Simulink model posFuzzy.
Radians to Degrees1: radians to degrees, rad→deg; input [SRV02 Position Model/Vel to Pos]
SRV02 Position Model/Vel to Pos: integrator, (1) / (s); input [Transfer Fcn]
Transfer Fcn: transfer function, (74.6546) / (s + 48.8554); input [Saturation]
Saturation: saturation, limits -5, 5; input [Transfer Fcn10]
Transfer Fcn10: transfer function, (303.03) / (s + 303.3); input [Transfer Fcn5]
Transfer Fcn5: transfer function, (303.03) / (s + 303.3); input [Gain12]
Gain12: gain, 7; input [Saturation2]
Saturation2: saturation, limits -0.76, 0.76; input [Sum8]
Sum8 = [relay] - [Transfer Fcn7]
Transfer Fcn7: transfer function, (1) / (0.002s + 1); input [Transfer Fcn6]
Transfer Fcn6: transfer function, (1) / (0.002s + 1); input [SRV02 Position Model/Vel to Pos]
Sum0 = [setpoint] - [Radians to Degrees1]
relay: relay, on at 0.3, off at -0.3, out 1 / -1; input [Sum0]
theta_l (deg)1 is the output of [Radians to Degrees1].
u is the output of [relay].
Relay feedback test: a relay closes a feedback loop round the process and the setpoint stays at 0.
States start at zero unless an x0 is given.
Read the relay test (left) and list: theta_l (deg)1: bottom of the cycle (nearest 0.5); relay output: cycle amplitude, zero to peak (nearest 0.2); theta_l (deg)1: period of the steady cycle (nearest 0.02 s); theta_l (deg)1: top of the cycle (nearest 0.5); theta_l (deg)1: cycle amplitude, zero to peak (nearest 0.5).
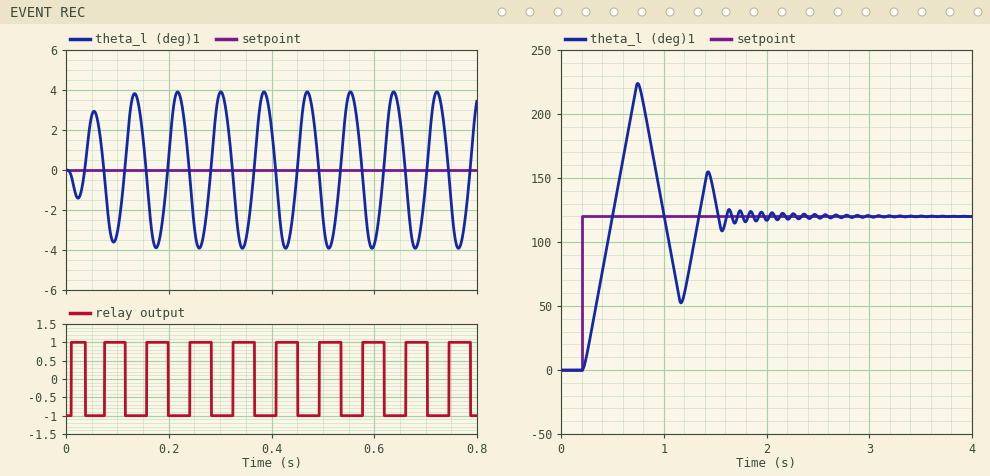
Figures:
-4.0
1.0
0.08 s
4.0
4.0
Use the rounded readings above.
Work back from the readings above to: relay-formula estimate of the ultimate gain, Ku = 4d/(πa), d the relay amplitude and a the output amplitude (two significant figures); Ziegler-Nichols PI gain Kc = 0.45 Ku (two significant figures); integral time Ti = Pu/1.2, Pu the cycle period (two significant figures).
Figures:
0.32
0.14
0.067 s
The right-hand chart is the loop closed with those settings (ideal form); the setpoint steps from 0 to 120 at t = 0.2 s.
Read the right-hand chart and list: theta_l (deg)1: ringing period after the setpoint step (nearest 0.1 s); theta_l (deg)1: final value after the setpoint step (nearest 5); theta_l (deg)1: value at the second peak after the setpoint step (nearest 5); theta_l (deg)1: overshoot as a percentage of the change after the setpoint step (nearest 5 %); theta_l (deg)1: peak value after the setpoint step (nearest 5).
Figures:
0.7 s
120
155
85 %
225
